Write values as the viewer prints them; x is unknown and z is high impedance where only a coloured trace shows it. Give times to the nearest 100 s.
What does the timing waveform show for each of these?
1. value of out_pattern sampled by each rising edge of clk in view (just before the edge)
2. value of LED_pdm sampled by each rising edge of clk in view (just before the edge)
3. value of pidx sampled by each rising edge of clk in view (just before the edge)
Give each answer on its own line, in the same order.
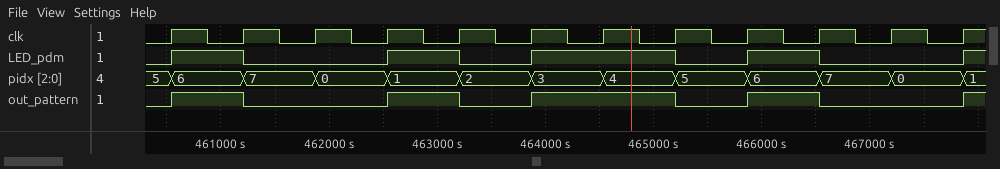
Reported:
0 1 0 0 1 0 1 1 0 1 0 0
0 1 0 0 1 0 1 1 0 1 0 0
5, 6, 7, 0, 1, 2, 3, 4, 5, 6, 7, 0
